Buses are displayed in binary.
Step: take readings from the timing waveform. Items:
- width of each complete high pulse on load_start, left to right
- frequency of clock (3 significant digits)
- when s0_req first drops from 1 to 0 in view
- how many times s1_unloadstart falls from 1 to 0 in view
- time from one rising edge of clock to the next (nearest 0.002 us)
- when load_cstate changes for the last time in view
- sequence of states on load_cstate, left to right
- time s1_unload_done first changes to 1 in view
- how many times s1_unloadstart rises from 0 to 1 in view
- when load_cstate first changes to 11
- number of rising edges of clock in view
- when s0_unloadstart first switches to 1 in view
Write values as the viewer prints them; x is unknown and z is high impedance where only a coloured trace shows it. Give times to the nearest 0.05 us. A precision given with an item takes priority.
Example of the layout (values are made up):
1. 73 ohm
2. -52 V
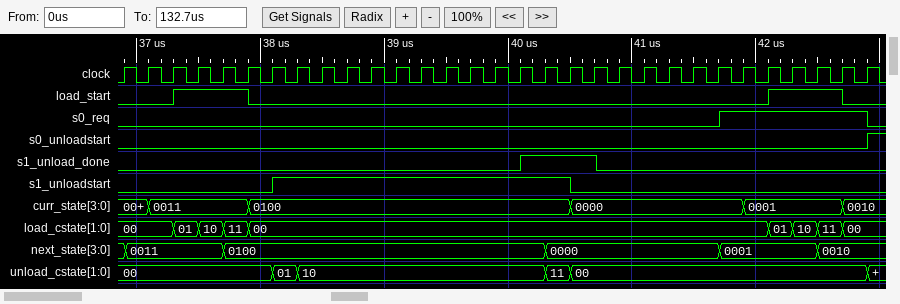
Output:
1. 0.6 us, 0.6 us
2. 5.00 MHz
3. 42.9 us
4. 1
5. 0.2 us
6. 42.7 us
7. 00, 01, 10, 11, 00, 01, 10, 11, 00
8. 40.1 us
9. 1
10. 37.7 us
11. 31
12. 42.9 us
